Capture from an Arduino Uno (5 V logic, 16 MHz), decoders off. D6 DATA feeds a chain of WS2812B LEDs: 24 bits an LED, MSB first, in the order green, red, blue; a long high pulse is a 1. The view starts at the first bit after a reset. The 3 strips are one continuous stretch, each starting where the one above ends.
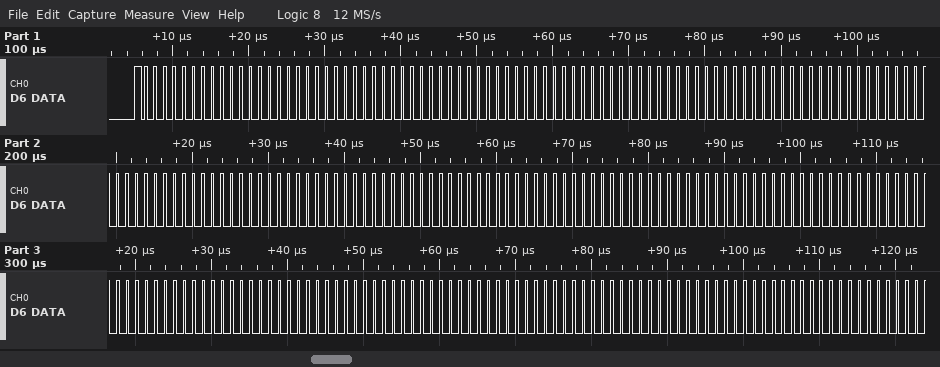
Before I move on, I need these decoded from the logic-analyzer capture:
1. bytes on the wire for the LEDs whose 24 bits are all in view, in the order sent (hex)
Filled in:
80 00 00 00 00 00 00 00 00 00 00 00 00 00 00 00 00 00 00 00 00 00 00 00 00 00 00 00 00 00
